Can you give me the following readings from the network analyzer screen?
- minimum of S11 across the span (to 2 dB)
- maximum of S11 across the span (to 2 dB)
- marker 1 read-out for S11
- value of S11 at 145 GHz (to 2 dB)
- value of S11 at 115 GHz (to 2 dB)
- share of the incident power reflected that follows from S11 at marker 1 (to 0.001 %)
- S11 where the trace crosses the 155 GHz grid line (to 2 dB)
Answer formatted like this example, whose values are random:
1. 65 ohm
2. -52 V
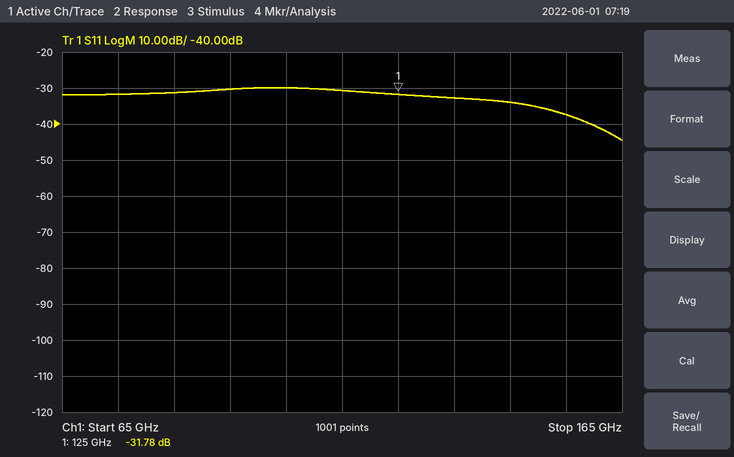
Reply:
1. -44 dB
2. -30 dB
3. -31.78 dB
4. -34 dB
5. -30 dB
6. 0.066 %
7. -38 dB
